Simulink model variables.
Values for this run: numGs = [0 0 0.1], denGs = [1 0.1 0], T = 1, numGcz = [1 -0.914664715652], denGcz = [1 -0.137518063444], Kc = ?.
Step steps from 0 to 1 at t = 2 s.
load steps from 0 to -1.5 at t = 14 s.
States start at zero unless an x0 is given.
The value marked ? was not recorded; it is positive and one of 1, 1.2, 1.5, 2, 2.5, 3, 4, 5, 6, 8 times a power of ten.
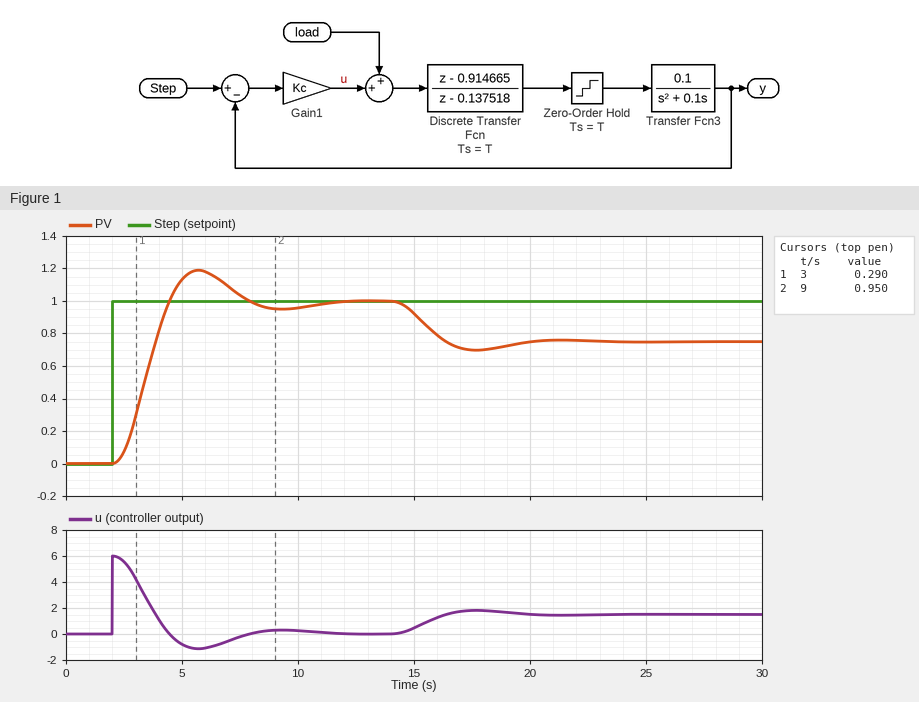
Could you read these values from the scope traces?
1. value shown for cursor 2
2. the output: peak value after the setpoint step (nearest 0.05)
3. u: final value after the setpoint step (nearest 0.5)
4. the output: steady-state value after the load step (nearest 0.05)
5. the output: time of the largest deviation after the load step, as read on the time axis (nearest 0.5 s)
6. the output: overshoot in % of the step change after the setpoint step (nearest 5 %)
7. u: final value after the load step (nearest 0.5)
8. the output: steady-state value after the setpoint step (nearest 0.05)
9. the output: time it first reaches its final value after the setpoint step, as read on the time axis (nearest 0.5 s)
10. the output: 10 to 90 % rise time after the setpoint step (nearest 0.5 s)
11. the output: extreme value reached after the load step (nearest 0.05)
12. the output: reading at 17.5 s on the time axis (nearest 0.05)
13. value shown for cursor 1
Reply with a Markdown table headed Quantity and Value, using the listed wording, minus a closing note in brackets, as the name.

| Quantity | Value |
|---|---|
| value shown for cursor 2 | 0.950 |
| the output: peak value after the setpoint step | 1.20 |
| u: final value after the setpoint step | 0.0 |
| the output: steady-state value after the load step | 0.75 |
| the output: time of the largest deviation after the load step, as read on the time axis | 17.5 s |
| the output: overshoot in % of the step change after the setpoint step | 20 % |
| u: final value after the load step | 1.5 |
| the output: steady-state value after the setpoint step | 1.00 |
| the output: time it first reaches its final value after the setpoint step, as read on the time axis | 4.5 s |
| the output: 10 to 90 % rise time after the setpoint step | 1.5 s |
| the output: extreme value reached after the load step | 0.70 |
| the output: reading at 17.5 s on the time axis | 0.70 |
| value shown for cursor 1 | 0.290 |
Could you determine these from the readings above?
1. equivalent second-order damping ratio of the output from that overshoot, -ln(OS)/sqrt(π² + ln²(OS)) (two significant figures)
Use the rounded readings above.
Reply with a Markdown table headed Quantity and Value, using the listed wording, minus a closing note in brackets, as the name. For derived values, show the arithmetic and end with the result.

| Quantity | Value |
|---|---|
| equivalent second-order damping ratio of the output from that overshoot, -ln(OS)/sqrt(π² + ln²(OS)) | ln(0.2) = -1.609; 1.609 / sqrt(9.870 + 2.590) = 0.46 |
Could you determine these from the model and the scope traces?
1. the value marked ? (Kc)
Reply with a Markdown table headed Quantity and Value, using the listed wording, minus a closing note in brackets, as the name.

| Quantity | Value |
|---|---|
| the value marked ? | 6 |
